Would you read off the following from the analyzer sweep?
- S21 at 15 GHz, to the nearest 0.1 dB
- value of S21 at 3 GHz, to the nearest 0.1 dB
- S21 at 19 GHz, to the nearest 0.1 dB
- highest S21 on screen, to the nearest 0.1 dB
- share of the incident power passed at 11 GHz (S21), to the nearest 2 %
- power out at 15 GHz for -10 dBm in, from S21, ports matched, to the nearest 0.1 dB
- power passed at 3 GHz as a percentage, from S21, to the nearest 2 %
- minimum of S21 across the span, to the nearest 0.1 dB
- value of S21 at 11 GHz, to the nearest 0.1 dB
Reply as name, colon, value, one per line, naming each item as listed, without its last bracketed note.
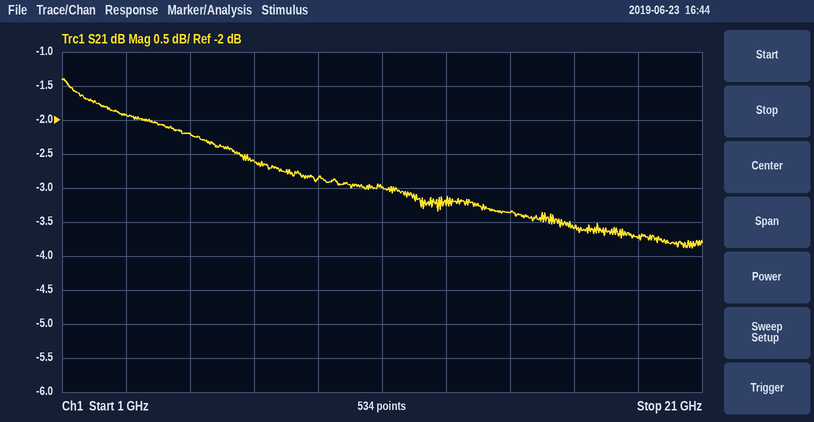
S21 at 15 GHz, to the nearest 0.1 dB: -3.4 dB
value of S21 at 3 GHz, to the nearest 0.1 dB: -1.9 dB
S21 at 19 GHz, to the nearest 0.1 dB: -3.7 dB
highest S21 on screen, to the nearest 0.1 dB: -1.4 dB
share of the incident power passed at 11 GHz (S21), to the nearest 2 %: 50 %
power out at 15 GHz for -10 dBm in, from S21, ports matched, to the nearest 0.1 dB: -13.4 dBm
power passed at 3 GHz as a percentage, from S21, to the nearest 2 %: 64 %
minimum of S21 across the span, to the nearest 0.1 dB: -3.9 dB
value of S21 at 11 GHz, to the nearest 0.1 dB: -3.0 dB
